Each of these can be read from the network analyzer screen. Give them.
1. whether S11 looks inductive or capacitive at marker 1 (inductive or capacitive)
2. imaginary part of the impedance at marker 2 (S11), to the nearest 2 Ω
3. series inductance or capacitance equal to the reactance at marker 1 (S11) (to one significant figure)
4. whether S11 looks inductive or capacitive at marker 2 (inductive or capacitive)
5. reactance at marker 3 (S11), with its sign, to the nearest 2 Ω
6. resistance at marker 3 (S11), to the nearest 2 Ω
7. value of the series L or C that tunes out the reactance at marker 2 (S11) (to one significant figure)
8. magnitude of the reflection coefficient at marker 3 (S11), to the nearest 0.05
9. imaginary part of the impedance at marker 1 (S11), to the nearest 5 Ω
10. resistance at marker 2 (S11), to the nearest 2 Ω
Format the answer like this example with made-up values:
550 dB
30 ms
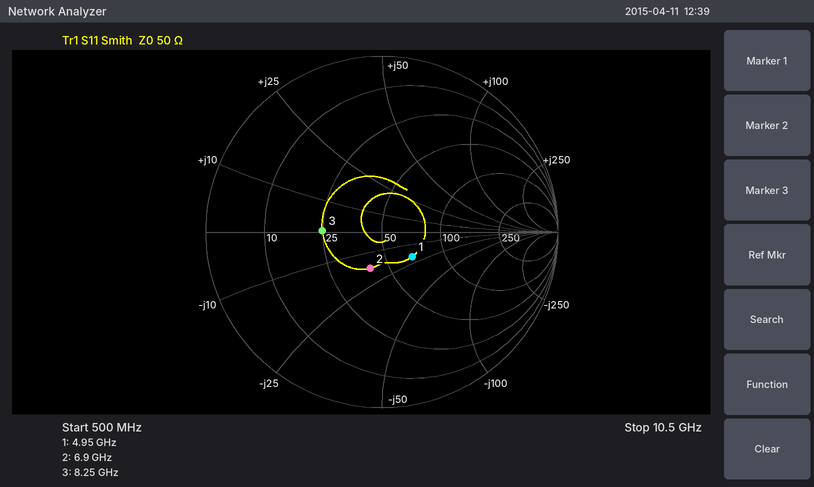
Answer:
capacitive
-18 Ω
2 pF
capacitive
0 Ω
24 Ω
400 pH
0.35
-20 Ω
40 Ω
